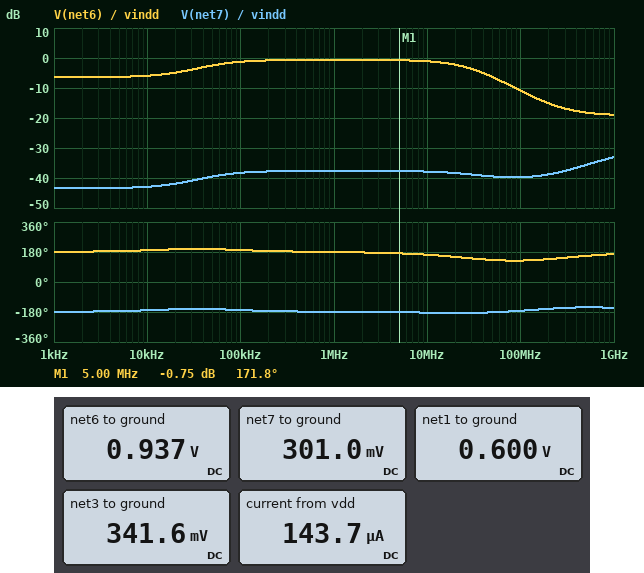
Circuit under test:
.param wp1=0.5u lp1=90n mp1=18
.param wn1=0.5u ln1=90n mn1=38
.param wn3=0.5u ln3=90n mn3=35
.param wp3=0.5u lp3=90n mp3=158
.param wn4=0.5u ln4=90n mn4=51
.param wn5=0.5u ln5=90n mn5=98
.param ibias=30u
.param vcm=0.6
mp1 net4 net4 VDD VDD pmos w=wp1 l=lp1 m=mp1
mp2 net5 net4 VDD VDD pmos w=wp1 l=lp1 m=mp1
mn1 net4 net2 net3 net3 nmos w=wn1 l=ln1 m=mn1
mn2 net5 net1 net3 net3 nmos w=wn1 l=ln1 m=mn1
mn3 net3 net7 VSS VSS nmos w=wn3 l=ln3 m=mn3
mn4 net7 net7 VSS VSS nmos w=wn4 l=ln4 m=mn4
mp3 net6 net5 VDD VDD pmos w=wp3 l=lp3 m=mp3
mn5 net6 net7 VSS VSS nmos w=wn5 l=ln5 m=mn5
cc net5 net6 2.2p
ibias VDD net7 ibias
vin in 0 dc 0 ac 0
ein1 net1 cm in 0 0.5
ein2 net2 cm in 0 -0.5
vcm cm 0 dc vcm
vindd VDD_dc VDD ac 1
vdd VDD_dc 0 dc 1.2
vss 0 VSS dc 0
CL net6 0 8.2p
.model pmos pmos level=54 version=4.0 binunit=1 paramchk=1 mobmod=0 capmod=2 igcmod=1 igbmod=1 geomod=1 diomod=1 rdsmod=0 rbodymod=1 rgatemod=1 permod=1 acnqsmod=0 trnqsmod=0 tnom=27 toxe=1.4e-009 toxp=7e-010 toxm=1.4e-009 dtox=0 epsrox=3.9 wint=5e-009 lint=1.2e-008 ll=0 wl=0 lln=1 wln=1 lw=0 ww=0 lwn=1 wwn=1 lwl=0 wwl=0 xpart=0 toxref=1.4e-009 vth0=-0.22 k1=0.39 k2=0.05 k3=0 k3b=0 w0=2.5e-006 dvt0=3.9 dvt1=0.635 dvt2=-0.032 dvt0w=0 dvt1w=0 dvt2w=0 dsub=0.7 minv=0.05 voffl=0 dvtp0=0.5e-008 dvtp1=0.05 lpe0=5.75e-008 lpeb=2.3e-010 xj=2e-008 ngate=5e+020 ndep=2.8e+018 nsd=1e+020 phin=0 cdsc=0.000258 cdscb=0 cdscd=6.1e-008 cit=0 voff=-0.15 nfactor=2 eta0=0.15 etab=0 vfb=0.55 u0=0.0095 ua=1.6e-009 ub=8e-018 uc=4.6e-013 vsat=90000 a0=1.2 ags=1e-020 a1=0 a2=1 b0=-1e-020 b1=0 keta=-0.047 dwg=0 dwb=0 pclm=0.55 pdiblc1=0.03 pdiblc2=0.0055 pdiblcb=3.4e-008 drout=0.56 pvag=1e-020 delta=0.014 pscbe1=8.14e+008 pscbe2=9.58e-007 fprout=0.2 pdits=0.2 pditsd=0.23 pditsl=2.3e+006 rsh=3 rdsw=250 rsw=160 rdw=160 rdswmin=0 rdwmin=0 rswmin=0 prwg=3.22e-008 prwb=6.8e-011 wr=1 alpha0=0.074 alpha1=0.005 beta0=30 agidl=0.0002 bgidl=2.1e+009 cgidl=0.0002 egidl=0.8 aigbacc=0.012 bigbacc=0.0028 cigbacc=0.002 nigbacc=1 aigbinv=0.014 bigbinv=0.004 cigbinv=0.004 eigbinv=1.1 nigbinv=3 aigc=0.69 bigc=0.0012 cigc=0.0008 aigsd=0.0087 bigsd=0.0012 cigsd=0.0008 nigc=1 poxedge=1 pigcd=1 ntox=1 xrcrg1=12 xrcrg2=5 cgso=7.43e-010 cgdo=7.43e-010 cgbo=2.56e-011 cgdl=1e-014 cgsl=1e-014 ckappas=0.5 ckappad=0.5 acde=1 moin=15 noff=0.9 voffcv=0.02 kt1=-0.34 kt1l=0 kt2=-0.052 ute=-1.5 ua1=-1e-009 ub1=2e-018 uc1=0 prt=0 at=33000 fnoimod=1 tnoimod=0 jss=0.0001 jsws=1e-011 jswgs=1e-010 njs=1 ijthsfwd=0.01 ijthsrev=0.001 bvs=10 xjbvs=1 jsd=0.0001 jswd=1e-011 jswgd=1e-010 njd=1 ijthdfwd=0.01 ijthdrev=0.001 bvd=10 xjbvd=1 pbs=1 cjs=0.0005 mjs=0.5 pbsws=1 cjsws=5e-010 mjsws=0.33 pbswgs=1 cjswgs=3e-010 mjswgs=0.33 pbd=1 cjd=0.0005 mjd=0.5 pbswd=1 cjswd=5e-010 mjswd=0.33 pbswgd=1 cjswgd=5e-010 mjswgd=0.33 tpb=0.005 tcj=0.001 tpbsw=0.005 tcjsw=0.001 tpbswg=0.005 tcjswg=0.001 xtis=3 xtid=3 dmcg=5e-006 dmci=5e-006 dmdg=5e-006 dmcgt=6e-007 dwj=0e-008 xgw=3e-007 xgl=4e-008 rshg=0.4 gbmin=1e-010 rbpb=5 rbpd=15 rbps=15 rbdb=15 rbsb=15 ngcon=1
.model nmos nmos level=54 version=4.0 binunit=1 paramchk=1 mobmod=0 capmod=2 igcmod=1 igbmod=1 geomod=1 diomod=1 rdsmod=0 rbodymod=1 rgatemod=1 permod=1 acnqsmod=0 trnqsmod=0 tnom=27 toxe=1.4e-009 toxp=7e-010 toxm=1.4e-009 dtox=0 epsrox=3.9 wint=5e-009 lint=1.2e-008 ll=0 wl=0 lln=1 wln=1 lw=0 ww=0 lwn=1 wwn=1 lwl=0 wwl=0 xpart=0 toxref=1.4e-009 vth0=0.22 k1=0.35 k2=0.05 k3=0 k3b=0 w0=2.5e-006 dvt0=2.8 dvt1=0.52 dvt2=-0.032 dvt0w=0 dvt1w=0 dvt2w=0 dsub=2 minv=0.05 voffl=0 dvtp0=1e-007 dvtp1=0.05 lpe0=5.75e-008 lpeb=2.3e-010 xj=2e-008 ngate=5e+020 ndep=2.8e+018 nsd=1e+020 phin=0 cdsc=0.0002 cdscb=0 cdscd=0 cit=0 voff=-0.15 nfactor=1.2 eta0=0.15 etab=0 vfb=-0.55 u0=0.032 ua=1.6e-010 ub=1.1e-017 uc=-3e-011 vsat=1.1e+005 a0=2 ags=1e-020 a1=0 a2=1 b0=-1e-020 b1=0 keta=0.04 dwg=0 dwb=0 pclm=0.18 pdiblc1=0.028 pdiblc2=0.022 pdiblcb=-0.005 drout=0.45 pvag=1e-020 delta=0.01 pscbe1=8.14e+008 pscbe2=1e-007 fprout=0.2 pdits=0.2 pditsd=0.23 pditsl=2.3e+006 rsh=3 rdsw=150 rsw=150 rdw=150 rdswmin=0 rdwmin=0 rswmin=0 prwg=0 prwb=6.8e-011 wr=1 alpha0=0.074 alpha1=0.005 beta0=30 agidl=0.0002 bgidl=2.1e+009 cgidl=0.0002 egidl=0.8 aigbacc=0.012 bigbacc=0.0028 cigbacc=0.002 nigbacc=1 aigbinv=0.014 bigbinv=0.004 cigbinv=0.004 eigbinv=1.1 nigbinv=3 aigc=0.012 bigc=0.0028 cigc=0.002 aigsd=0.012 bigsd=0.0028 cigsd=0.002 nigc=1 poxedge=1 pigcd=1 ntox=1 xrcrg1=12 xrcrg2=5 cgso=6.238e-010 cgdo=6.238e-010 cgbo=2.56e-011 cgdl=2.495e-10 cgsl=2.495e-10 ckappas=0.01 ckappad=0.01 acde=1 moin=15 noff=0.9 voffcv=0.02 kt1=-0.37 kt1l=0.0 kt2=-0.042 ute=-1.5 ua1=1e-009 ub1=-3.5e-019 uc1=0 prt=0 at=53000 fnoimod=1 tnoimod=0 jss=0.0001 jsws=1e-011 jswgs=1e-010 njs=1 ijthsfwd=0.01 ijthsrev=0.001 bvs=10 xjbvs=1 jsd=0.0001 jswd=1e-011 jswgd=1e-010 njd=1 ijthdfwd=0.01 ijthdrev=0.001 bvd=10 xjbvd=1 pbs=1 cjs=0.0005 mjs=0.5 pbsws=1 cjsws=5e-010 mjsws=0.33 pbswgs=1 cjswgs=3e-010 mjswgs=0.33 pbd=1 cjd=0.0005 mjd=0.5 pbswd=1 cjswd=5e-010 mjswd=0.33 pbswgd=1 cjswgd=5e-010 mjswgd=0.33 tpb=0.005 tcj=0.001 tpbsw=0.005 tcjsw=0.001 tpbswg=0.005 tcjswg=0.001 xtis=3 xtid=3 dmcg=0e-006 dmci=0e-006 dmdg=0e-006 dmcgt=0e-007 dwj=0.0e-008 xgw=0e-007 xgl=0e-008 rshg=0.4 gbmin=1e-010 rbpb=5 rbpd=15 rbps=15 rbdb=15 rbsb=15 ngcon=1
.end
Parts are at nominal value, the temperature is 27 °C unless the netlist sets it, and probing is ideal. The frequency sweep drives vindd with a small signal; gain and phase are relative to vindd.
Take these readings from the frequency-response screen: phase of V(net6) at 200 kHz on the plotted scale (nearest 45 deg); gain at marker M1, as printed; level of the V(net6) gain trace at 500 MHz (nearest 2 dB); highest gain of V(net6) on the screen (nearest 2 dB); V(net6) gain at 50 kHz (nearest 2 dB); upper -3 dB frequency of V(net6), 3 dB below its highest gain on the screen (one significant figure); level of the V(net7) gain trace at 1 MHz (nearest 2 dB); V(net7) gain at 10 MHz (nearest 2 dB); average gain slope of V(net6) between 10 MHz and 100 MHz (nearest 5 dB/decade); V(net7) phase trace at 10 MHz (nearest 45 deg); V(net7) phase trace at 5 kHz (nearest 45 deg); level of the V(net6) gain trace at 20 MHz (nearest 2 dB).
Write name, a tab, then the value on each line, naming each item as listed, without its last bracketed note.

phase of V(net6) at 200 kHz on the plotted scale	180 deg
gain at marker M1, as printed	-0.75 dB
level of the V(net6) gain trace at 500 MHz	-18 dB
highest gain of V(net6) on the screen	0 dB
V(net6) gain at 50 kHz	-2 dB
upper -3 dB frequency of V(net6), 3 dB below its highest gain on the screen	30 MHz
level of the V(net7) gain trace at 1 MHz	-38 dB
V(net7) gain at 10 MHz	-38 dB
average gain slope of V(net6) between 10 MHz and 100 MHz	-10 dB/decade
V(net7) phase trace at 10 MHz	-180 deg
V(net7) phase trace at 5 kHz	-180 deg
level of the V(net6) gain trace at 20 MHz	-2 dB
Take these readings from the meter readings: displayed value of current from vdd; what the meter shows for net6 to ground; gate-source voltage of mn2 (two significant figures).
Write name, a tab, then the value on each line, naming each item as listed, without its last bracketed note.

displayed value of current from vdd	143.7 µA
what the meter shows for net6 to ground	0.937 V
gate-source voltage of mn2	260 mV
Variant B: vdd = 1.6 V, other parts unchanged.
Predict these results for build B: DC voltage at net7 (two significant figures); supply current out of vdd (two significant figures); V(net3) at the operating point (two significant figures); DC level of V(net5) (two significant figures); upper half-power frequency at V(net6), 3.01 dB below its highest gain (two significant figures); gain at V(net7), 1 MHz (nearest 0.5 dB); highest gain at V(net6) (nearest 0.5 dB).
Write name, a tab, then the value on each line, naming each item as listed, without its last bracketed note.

DC voltage at net7	310 mV
supply current out of vdd	170 µA
V(net3) at the operating point	350 mV
DC level of V(net5)	1.3 V
upper half-power frequency at V(net6), 3.01 dB below its highest gain	38 MHz
gain at V(net7), 1 MHz	-30.0 dB
highest gain at V(net6)	-1.0 dB
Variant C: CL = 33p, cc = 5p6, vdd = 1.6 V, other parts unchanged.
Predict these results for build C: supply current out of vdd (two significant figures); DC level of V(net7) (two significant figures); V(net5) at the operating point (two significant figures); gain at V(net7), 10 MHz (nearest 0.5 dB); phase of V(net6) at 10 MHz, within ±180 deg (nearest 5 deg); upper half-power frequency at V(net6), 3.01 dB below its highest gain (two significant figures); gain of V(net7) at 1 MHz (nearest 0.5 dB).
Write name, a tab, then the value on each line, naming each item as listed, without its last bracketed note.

supply current out of vdd	170 µA
DC level of V(net7)	310 mV
V(net5) at the operating point	1.3 V
gain at V(net7), 10 MHz	-32.5 dB
phase of V(net6) at 10 MHz, within ±180 deg	140 deg
upper half-power frequency at V(net6), 3.01 dB below its highest gain	11 MHz
gain of V(net7) at 1 MHz	-30.0 dB
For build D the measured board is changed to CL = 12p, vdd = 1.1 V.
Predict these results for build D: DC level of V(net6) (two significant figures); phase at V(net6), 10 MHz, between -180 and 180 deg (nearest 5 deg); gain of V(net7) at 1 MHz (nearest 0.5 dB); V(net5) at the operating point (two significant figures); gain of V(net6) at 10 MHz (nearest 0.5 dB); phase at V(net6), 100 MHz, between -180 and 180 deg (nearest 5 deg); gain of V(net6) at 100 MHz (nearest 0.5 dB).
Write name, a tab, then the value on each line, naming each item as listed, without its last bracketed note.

DC level of V(net6)	890 mV
phase at V(net6), 10 MHz, between -180 and 180 deg	155 deg
gain of V(net7) at 1 MHz	-40.0 dB
V(net5) at the operating point	770 mV
gain of V(net6) at 10 MHz	-1.5 dB
phase at V(net6), 100 MHz, between -180 and 180 deg	125 deg
gain of V(net6) at 100 MHz	-14.0 dB
